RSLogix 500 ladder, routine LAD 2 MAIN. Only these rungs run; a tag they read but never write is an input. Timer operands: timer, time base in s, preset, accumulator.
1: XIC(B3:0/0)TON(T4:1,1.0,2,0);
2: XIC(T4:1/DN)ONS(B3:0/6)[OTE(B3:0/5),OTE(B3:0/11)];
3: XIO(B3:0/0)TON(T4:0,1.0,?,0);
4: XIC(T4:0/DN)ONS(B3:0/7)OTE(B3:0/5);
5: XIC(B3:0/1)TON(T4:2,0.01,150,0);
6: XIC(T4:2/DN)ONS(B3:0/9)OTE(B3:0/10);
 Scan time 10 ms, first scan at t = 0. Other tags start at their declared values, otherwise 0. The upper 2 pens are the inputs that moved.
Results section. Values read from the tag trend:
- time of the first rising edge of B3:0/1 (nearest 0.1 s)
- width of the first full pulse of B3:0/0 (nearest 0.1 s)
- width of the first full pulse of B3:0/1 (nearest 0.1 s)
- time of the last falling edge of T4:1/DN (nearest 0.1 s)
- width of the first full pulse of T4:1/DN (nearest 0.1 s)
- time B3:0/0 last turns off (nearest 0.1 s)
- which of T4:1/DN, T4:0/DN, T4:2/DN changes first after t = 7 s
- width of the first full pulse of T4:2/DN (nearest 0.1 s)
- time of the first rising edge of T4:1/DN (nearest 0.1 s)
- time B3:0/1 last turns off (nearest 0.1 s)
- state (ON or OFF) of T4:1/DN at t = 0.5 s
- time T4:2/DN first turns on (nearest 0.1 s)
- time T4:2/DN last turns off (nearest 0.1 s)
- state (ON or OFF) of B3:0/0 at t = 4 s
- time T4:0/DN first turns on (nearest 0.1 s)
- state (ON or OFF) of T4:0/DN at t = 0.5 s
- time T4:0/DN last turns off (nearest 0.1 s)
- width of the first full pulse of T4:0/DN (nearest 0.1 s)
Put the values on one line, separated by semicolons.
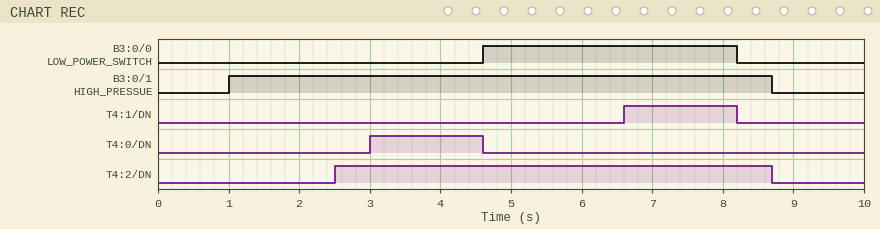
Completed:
1.0 s; 3.6 s; 7.7 s; 8.2 s; 1.6 s; 8.2 s; T4:1/DN; 6.2 s; 6.6 s; 8.7 s; OFF; 2.5 s; 8.7 s; OFF; 3.0 s; OFF; 4.6 s; 1.6 s
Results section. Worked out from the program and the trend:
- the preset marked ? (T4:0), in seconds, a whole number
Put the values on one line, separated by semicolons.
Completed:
3 s
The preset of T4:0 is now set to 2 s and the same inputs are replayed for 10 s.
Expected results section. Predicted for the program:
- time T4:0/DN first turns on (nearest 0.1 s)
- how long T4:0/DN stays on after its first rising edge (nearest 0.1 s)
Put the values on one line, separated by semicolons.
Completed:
2.0 s; 2.6 s
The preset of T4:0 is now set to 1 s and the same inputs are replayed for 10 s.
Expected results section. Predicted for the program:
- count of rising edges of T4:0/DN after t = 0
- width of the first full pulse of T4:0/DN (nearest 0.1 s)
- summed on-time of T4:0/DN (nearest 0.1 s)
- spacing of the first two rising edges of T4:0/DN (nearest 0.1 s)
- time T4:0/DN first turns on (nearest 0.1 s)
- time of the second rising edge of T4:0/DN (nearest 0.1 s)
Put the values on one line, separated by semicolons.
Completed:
2; 3.6 s; 4.4 s; 8.2 s; 1.0 s; 9.2 s
